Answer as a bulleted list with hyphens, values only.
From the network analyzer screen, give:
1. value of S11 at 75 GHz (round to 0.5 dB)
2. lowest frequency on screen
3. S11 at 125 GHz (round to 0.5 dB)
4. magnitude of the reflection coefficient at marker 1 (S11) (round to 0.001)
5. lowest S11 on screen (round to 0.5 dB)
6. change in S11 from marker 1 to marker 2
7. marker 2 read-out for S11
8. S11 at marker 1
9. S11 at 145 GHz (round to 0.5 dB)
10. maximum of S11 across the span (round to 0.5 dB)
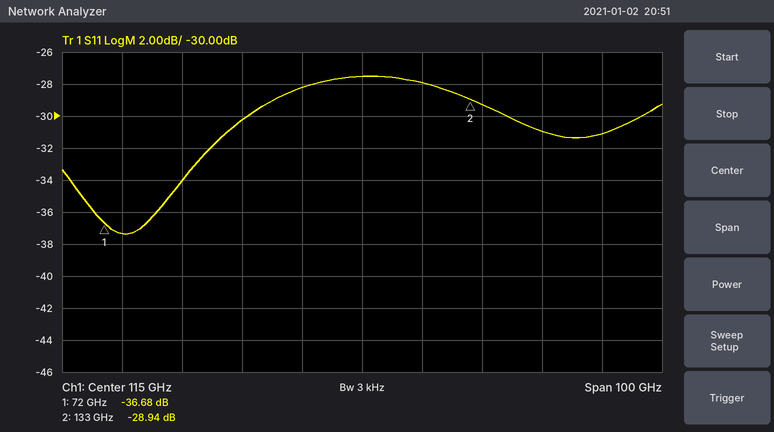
- -37.5 dB
- 65 GHz
- -28.0 dB
- 0.015
- -37.5 dB
- 7.74 dB
- -28.94 dB
- -36.68 dB
- -31.0 dB
- -27.5 dB
